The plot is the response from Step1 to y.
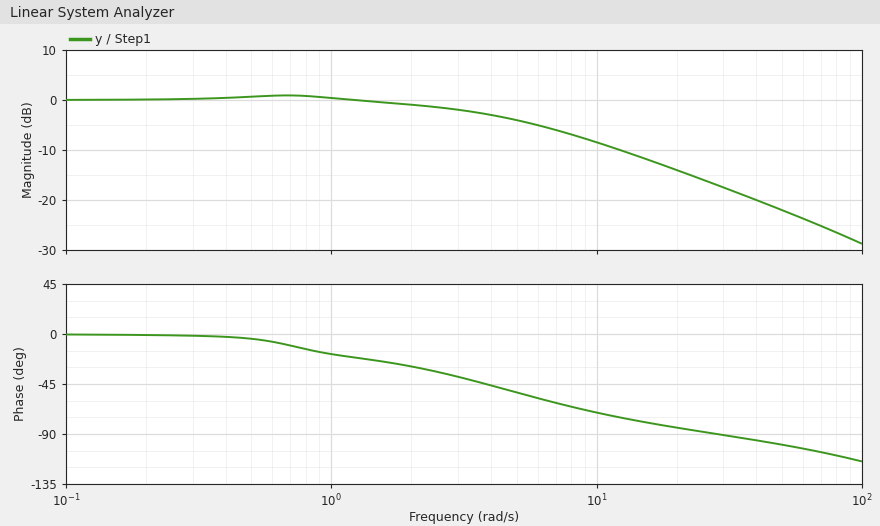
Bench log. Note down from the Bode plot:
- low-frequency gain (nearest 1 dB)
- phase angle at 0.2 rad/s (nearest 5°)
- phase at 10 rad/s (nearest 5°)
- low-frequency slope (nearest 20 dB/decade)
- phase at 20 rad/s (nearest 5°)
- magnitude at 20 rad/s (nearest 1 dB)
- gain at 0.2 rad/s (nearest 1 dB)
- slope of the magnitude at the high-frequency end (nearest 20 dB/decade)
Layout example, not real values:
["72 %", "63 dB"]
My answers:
["0 dB", "0°", "-70°", "0 dB/decade", "-85°", "-14 dB", "0 dB", "-20 dB/decade"]
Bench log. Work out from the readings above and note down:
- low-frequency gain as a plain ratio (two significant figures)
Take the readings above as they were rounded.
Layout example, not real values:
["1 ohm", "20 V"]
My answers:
["1.0"]
